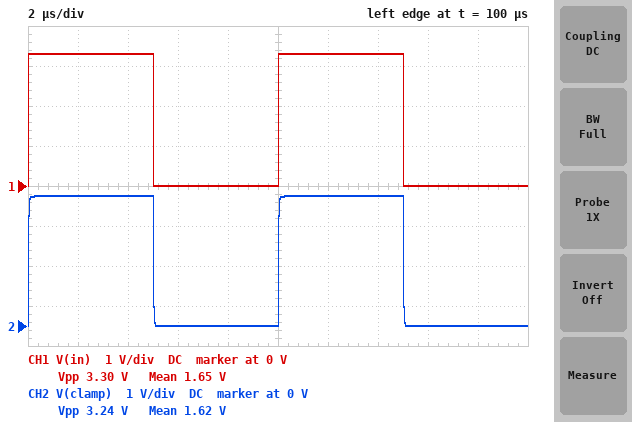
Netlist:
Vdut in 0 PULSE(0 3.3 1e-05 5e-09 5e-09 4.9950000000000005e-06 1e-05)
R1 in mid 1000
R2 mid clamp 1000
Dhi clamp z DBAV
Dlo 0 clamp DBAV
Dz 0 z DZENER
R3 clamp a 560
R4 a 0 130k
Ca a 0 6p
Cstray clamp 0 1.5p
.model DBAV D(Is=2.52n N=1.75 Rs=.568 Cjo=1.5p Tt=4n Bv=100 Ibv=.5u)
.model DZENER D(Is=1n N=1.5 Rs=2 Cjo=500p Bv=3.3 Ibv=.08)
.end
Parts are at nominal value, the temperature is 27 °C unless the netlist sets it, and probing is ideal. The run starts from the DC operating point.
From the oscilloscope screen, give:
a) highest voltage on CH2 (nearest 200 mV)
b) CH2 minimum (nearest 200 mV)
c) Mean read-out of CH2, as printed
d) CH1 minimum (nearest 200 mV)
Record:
3.2 V
0 V
1.62 V
0 V
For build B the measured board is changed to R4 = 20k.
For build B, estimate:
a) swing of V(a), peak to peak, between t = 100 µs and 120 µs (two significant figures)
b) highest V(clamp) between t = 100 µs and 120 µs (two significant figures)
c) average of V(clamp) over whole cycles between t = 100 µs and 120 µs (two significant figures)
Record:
2.9 V
3.0 V
1.5 V
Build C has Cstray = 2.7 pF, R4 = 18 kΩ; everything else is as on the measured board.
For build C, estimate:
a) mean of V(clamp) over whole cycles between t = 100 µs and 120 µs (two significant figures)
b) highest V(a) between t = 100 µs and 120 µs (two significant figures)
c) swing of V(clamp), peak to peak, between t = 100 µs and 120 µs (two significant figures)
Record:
1.5 V
2.9 V
3.0 V
